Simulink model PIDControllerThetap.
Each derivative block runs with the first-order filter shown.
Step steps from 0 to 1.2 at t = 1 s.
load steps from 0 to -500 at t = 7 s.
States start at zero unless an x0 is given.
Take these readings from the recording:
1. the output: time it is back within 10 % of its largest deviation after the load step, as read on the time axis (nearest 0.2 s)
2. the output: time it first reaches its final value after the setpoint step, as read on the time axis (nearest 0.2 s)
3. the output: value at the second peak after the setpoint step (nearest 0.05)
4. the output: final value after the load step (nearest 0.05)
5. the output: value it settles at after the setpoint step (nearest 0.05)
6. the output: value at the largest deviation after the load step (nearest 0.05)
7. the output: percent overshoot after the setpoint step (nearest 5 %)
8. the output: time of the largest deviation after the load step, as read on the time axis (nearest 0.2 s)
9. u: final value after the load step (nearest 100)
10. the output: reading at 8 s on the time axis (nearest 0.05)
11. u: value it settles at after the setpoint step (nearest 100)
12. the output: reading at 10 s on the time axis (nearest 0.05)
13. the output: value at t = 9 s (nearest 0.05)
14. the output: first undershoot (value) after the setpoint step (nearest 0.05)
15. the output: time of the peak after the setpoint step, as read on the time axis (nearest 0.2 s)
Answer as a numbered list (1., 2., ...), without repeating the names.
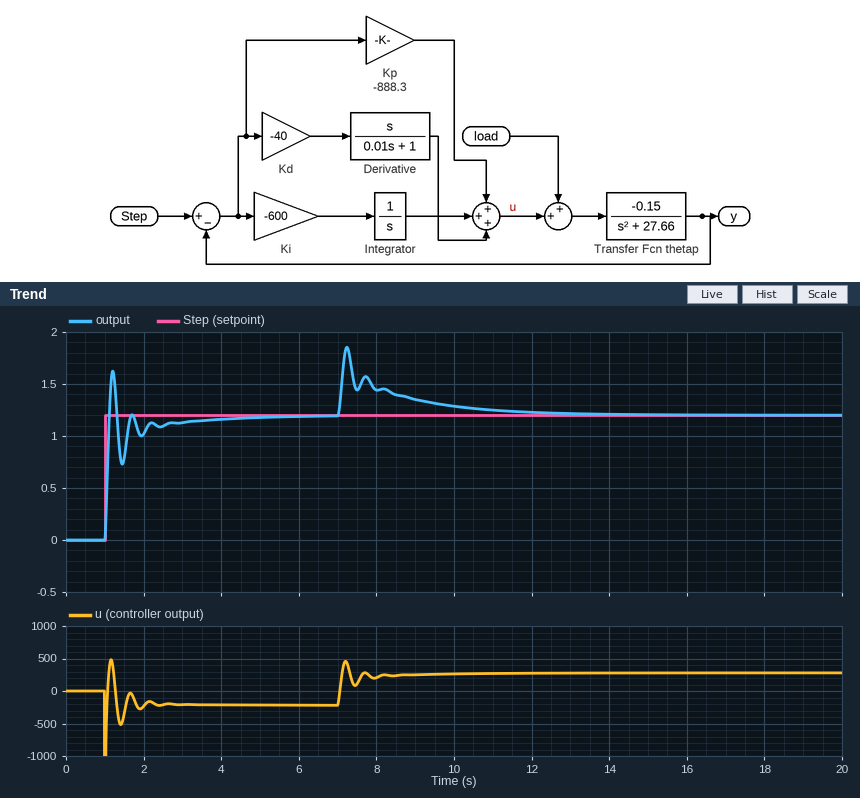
1. 10.4 s
2. 1.2 s
3. 1.20
4. 1.20
5. 1.20
6. 1.85
7. 35 %
8. 7.2 s
9. 300
10. 1.45
11. -200
12. 1.30
13. 1.35
14. 0.75
15. 1.2 s
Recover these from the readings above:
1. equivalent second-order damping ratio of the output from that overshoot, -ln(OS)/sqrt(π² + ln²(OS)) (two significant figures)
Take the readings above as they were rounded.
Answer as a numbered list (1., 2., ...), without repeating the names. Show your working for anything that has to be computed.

1. ln(0.35) = -1.050; 1.050 / sqrt(9.870 + 1.102) = 0.32
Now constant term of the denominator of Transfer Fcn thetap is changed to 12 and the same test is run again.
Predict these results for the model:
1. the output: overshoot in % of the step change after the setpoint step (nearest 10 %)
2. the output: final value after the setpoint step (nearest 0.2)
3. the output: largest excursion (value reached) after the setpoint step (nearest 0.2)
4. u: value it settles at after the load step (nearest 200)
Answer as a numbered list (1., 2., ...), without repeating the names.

1. 50 %
2. 1.2
3. 1.8
4. 400
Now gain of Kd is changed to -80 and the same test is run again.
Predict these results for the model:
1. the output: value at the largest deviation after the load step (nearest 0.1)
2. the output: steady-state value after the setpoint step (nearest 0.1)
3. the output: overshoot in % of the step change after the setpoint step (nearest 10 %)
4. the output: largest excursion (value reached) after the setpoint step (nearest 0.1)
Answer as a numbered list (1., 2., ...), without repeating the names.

1. 1.7
2. 1.2
3. 20 %
4. 1.4
